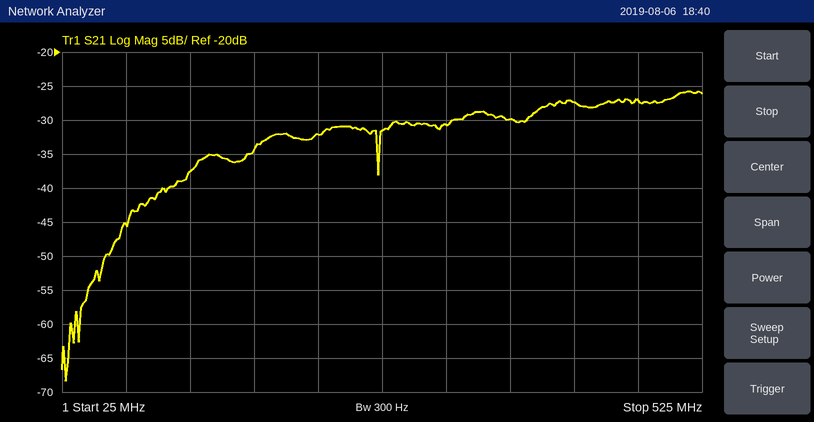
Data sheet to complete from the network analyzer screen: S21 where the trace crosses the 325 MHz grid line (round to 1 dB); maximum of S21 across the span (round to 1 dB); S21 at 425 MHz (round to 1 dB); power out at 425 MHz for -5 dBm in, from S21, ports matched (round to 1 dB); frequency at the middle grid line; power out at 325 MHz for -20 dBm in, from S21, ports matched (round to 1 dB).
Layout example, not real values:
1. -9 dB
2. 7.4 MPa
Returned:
1. -31 dB
2. -26 dB
3. -27 dB
4. -32 dBm
5. 275 MHz
6. -51 dBm
